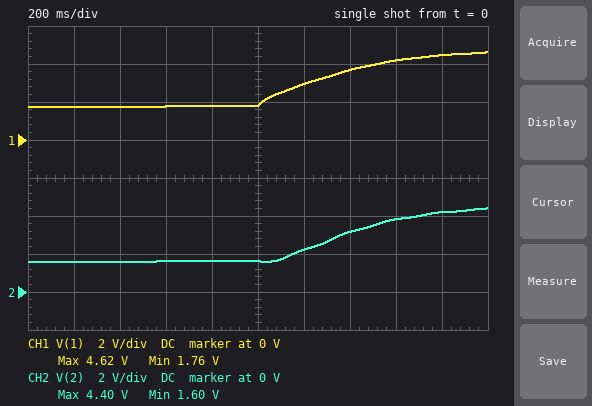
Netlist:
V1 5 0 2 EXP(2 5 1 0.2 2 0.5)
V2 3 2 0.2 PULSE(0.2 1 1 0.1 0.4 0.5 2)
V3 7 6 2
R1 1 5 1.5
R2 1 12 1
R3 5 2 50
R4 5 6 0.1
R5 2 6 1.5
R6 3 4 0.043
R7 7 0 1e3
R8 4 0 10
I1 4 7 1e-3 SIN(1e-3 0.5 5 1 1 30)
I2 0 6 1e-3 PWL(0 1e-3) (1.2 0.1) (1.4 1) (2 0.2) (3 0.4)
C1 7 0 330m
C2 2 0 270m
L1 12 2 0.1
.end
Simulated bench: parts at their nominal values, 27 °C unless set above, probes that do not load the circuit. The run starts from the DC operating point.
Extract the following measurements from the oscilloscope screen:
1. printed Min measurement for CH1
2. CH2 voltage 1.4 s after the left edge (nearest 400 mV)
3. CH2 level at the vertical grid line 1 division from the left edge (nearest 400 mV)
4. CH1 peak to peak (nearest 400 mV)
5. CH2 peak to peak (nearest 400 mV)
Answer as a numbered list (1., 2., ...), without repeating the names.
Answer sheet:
1. 1.76 V
2. 3.2 V
3. 1.6 V
4. 2.8 V
5. 2.8 V
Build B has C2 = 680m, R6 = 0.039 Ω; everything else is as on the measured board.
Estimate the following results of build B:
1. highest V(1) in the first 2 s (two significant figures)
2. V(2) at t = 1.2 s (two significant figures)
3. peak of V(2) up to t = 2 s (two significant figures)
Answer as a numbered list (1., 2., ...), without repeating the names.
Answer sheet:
1. 4.2 V
2. 1.9 V
3. 3.7 V
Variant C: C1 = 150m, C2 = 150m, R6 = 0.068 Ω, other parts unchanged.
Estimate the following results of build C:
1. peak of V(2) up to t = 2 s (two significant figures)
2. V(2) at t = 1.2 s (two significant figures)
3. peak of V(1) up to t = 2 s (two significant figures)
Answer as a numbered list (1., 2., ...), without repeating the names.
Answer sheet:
1. 4.5 V
2. 2.6 V
3. 4.7 V
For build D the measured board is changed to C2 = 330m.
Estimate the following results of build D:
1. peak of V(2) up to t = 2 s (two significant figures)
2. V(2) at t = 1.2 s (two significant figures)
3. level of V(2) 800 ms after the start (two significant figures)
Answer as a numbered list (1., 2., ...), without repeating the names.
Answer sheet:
1. 4.3 V
2. 2.1 V
3. 1.6 V
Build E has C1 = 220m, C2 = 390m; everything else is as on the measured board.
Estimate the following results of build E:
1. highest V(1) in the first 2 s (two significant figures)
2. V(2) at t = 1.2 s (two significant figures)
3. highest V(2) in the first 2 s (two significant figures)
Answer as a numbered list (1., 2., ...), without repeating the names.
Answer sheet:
1. 4.5 V
2. 2.1 V
3. 4.2 V
